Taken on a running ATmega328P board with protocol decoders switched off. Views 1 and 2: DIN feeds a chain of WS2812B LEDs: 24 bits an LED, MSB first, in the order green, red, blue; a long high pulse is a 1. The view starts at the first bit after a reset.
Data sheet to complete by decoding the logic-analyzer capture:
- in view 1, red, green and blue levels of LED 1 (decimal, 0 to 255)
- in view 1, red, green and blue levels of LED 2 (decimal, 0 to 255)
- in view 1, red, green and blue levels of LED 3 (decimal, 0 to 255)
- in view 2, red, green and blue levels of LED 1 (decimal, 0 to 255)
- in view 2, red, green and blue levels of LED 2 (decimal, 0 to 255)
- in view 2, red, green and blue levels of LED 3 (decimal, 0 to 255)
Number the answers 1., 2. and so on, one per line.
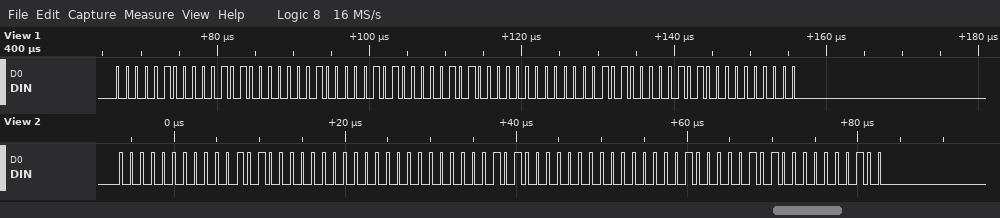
1. 20, 4, 4
2. 20, 20, 0
3. 20, 20, 0
4. 20, 0, 0
5. 20, 0, 0
6. 20, 4, 4
